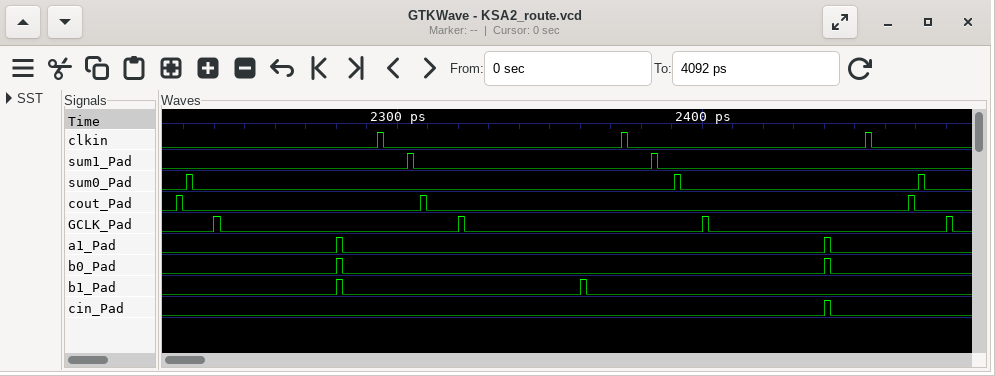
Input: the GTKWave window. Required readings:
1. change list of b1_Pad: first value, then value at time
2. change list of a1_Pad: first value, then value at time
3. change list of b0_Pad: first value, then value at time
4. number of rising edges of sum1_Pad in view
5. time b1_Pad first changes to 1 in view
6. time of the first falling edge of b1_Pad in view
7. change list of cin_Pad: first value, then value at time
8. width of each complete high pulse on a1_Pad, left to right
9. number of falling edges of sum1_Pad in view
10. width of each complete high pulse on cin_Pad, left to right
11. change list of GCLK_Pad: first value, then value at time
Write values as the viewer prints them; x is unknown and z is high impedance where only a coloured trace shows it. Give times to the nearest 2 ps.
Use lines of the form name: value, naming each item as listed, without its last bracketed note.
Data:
change list of b1_Pad: first value, then value at time: 0, 1 at 2280 ps, 0 at 2282 ps, 1 at 2360 ps, 0 at 2362 ps
change list of a1_Pad: first value, then value at time: 0, 1 at 2280 ps, 0 at 2282 ps, 1 at 2440 ps, 0 at 2442 ps
change list of b0_Pad: first value, then value at time: 0, 1 at 2280 ps, 0 at 2282 ps, 1 at 2440 ps, 0 at 2442 ps
number of rising edges of sum1_Pad in view: 2
time b1_Pad first changes to 1 in view: 2280 ps
time of the first falling edge of b1_Pad in view: 2282 ps
change list of cin_Pad: first value, then value at time: 0, 1 at 2440 ps, 0 at 2442 ps
width of each complete high pulse on a1_Pad, left to right: 2 ps, 2 ps
number of falling edges of sum1_Pad in view: 2
width of each complete high pulse on cin_Pad, left to right: 2 ps
change list of GCLK_Pad: first value, then value at time: 0, 1 at 2240 ps, 0 at 2242 ps, 1 at 2320 ps, 0 at 2322 ps, 1 at 2400 ps, 0 at 2402 ps, 1 at 2480 ps, 0 at 2482 ps
